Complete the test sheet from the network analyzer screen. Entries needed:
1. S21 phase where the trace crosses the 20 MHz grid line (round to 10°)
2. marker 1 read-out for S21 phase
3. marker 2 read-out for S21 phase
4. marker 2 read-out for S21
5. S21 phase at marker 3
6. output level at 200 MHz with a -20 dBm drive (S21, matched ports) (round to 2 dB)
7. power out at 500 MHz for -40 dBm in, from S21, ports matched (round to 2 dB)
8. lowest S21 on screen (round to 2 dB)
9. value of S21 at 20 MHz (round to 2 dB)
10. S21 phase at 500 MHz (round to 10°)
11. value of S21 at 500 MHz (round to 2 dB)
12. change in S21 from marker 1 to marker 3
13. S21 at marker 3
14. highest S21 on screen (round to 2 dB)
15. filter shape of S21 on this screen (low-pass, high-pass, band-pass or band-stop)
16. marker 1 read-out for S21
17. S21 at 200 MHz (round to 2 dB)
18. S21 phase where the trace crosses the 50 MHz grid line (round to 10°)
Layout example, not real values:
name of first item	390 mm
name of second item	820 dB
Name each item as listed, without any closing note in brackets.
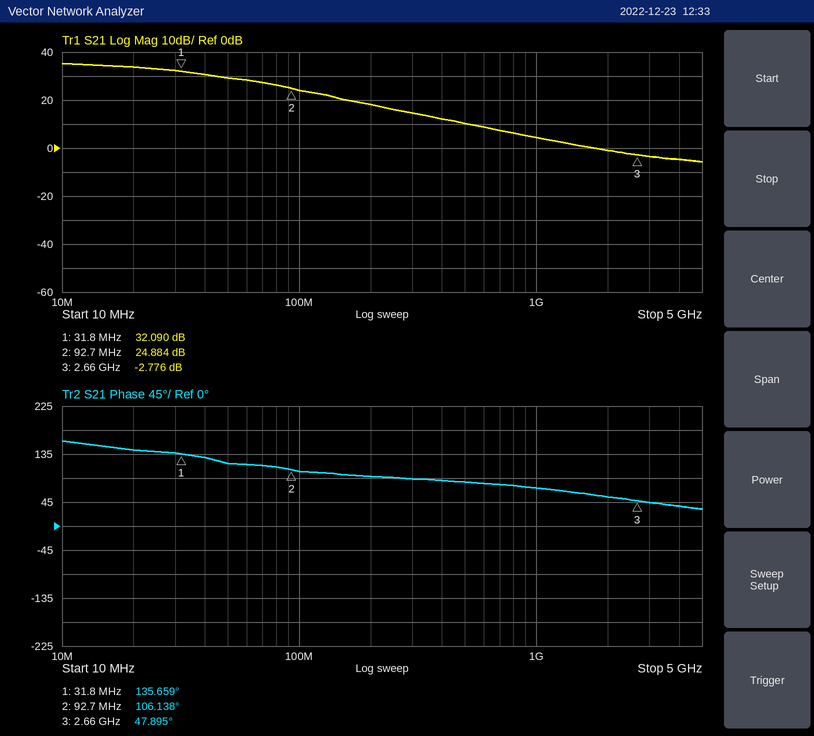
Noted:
S21 phase where the trace crosses the 20 MHz grid line	140°
marker 1 read-out for S21 phase	135.659°
marker 2 read-out for S21 phase	106.138°
marker 2 read-out for S21	24.884 dB
S21 phase at marker 3	47.895°
output level at 200 MHz with a -20 dBm drive (S21, matched ports)	-2 dBm
power out at 500 MHz for -40 dBm in, from S21, ports matched	-30 dBm
lowest S21 on screen	-6 dB
value of S21 at 20 MHz	34 dB
S21 phase at 500 MHz	80°
value of S21 at 500 MHz	10 dB
change in S21 from marker 1 to marker 3	-34.866 dB
S21 at marker 3	-2.776 dB
highest S21 on screen	36 dB
filter shape of S21 on this screen	low-pass
marker 1 read-out for S21	32.090 dB
S21 at 200 MHz	18 dB
S21 phase where the trace crosses the 50 MHz grid line	120°
